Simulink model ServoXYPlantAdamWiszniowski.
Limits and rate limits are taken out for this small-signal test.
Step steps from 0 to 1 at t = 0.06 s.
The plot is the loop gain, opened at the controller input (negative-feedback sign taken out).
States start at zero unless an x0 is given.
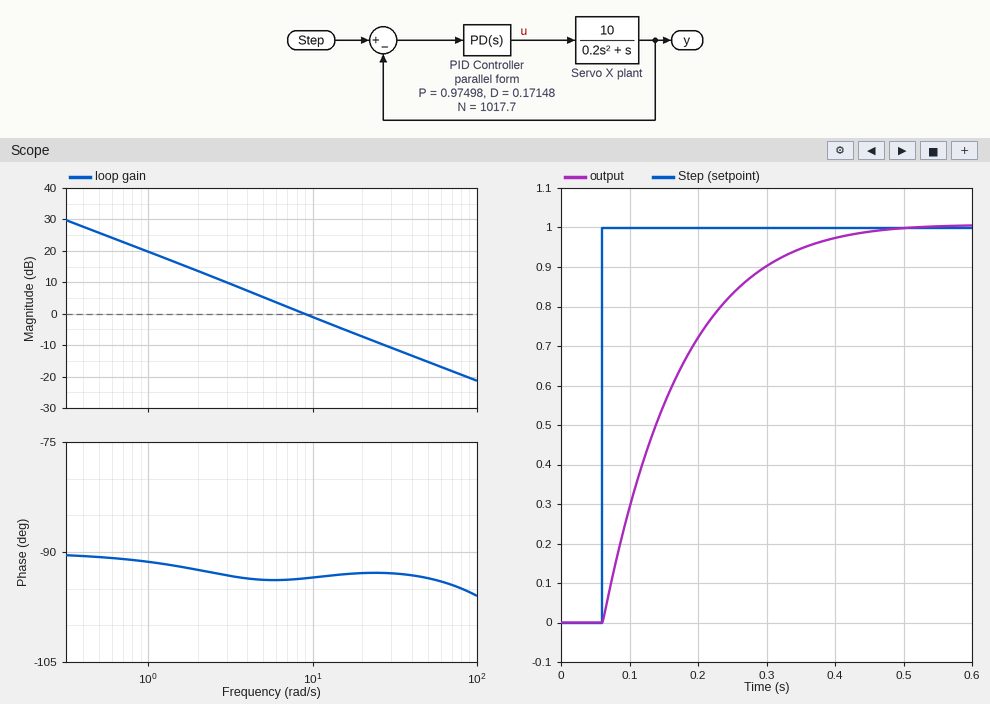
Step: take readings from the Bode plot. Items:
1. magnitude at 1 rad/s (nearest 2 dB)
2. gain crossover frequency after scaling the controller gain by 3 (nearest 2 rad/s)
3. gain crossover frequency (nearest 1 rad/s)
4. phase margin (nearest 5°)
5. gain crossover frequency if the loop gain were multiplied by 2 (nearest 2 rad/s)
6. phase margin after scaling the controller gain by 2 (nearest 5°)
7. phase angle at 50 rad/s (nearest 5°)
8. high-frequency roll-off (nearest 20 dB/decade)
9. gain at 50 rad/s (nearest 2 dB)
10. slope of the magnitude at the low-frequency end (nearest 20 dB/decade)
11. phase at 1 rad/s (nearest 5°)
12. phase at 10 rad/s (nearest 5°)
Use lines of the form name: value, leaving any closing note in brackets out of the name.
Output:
magnitude at 1 rad/s: 20 dB
gain crossover frequency after scaling the controller gain by 3: 26 rad/s
gain crossover frequency: 9 rad/s
phase margin: 85°
gain crossover frequency if the loop gain were multiplied by 2: 18 rad/s
phase margin after scaling the controller gain by 2: 85°
phase angle at 50 rad/s: -95°
high-frequency roll-off: -20 dB/decade
gain at 50 rad/s: -16 dB
slope of the magnitude at the low-frequency end: -20 dB/decade
phase at 1 rad/s: -90°
phase at 10 rad/s: -95°
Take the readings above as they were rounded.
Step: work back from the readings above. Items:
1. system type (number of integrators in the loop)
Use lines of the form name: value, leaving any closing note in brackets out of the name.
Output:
system type: 1
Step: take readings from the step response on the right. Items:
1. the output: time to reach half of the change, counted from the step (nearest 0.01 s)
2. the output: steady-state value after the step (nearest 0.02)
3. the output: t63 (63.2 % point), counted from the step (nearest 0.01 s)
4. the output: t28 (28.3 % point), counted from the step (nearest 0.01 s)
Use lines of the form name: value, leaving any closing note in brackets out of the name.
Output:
the output: time to reach half of the change, counted from the step: 0.08 s
the output: steady-state value after the step: 1.00
the output: t63 (63.2 % point), counted from the step: 0.11 s
the output: t28 (28.3 % point), counted from the step: 0.04 s
